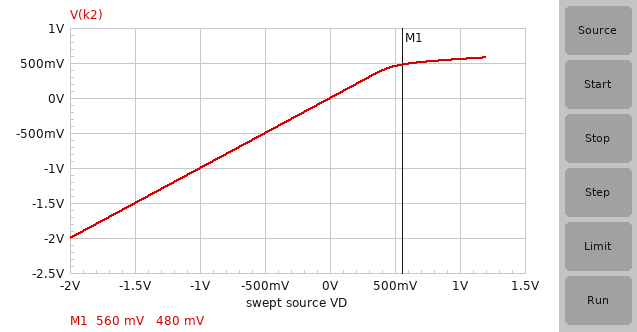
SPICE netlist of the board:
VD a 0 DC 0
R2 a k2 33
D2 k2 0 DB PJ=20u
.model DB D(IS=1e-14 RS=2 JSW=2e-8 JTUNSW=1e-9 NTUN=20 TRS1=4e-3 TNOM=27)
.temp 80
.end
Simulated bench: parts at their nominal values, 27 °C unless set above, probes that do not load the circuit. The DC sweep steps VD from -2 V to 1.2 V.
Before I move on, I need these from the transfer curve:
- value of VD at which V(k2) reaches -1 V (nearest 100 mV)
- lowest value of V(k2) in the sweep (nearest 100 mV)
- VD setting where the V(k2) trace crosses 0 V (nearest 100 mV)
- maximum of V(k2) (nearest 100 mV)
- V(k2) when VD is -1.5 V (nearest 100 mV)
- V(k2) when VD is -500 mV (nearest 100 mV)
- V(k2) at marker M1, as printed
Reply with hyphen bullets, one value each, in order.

- -1.0 V
- -2.0 V
- 0 V
- 600 mV
- -1.5 V
- -500 mV
- 480 mV
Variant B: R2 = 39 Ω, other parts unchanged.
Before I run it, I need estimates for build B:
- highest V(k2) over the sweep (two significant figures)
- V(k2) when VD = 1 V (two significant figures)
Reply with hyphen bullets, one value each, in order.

- 570 mV
- 550 mV
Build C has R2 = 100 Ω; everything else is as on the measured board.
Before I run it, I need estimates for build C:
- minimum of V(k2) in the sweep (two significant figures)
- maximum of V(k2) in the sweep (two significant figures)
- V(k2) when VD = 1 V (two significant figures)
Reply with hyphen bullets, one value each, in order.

- -2.0 V
- 520 mV
- 510 mV
